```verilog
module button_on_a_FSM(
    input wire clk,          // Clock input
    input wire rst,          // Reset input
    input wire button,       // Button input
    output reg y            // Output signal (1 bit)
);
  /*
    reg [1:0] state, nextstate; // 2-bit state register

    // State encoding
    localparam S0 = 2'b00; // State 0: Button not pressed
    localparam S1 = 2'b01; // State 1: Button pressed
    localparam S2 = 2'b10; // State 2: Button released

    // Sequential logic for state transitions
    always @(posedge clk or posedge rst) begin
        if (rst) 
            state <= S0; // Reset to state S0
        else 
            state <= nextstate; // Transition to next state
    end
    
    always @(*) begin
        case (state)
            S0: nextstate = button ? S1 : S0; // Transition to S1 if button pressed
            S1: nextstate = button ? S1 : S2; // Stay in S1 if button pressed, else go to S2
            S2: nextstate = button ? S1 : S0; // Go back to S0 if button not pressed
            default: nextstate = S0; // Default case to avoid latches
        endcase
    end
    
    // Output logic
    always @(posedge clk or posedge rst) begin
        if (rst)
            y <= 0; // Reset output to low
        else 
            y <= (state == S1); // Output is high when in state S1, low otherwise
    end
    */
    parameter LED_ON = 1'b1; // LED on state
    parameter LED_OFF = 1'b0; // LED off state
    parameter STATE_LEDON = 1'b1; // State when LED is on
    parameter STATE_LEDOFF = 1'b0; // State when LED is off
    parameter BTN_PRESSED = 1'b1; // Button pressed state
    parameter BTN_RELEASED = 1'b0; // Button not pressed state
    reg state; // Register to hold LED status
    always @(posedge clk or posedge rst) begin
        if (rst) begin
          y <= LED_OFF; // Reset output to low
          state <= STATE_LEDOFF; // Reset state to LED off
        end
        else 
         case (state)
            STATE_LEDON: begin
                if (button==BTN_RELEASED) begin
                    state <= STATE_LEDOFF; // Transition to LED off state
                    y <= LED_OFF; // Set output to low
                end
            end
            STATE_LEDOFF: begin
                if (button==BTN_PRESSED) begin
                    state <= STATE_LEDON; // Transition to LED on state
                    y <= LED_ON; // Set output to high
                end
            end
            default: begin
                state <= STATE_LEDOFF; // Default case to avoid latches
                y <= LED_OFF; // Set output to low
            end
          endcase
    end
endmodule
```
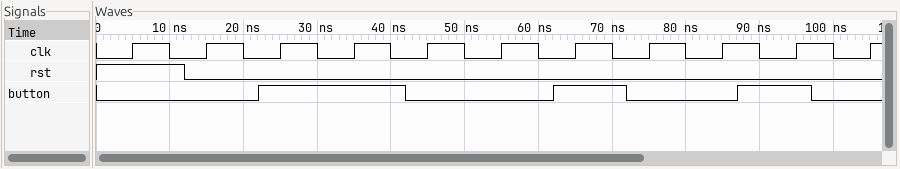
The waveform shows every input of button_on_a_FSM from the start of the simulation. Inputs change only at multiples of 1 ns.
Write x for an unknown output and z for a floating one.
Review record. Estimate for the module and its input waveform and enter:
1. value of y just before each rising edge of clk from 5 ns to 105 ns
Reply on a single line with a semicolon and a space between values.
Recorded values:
0 0 0 1 1 0 0 1 0 0 1
